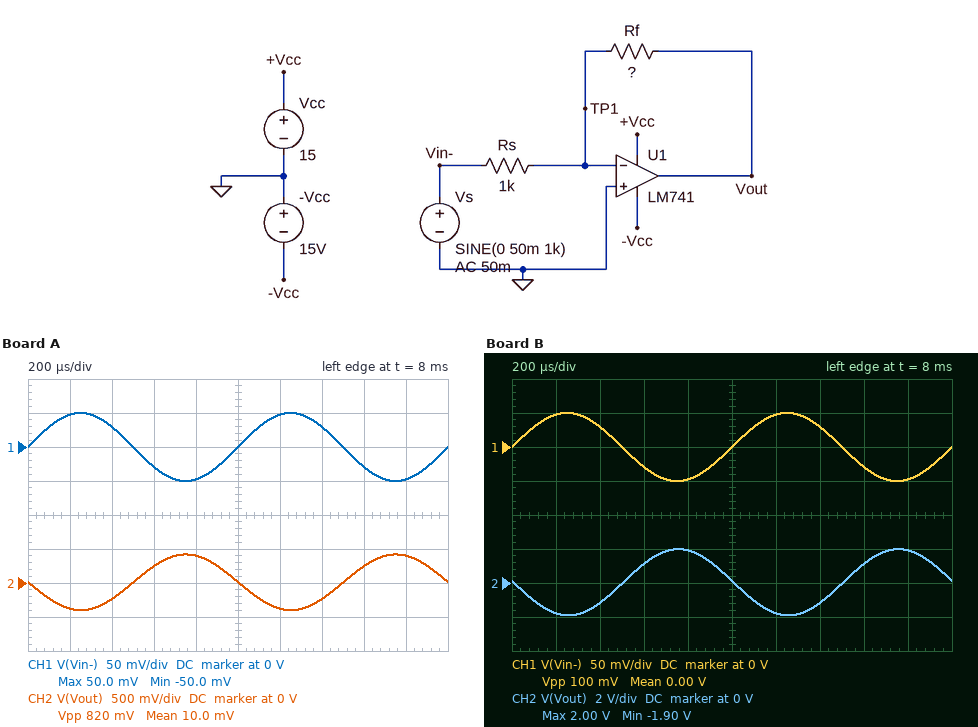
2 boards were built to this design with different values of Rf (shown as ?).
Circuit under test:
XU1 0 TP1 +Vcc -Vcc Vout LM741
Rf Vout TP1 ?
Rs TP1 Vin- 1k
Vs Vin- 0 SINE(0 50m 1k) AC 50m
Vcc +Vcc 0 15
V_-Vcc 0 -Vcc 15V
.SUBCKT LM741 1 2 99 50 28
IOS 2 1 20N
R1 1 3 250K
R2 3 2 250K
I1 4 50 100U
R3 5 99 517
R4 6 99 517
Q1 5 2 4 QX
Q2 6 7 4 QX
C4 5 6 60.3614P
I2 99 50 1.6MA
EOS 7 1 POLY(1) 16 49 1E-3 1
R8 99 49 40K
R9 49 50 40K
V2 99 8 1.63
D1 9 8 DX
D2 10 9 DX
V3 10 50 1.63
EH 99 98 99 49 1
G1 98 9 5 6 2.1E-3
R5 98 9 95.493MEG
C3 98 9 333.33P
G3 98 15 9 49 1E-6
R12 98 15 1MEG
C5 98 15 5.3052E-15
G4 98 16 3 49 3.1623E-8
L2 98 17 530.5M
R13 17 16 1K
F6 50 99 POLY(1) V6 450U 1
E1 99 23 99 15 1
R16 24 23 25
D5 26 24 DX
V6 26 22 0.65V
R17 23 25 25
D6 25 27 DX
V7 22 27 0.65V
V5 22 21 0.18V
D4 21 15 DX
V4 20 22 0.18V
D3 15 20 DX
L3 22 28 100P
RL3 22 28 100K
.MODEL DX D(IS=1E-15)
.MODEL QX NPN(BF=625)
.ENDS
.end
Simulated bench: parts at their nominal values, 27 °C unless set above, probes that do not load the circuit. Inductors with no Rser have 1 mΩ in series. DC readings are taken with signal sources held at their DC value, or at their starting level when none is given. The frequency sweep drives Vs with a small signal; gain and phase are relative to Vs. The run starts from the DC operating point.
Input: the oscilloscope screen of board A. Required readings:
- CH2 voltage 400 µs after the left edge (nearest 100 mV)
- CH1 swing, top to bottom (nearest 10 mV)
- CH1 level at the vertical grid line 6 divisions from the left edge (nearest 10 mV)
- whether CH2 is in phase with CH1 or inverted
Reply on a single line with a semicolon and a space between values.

-200 mV; 100 mV; 50 mV; inverted
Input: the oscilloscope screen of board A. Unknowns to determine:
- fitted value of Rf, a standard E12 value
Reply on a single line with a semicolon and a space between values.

8.2 kΩ
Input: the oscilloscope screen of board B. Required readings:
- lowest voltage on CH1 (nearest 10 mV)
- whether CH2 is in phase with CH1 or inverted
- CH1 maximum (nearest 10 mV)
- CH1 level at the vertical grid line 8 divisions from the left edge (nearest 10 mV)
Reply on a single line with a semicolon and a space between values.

-50 mV; inverted; 50 mV; -30 mV
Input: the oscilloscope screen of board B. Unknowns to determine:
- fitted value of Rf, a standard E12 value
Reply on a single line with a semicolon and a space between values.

39 kΩ
